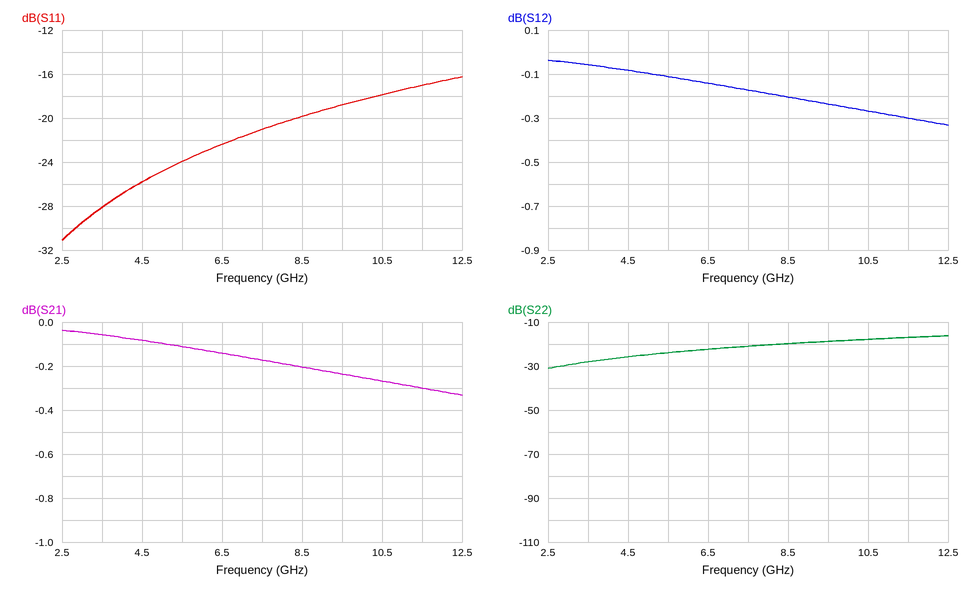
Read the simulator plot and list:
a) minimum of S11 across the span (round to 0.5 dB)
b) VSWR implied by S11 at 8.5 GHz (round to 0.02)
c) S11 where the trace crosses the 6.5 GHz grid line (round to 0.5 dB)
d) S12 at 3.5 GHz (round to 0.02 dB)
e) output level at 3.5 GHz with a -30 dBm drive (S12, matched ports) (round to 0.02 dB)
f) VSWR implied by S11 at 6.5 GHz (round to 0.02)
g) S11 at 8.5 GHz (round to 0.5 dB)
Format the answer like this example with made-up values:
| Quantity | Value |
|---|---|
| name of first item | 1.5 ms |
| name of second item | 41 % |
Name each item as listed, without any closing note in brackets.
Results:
| Quantity | Value |
|---|---|
| minimum of S11 across the span | -31.0 dB |
| VSWR implied by S11 at 8.5 GHz | 1.22 |
| S11 where the trace crosses the 6.5 GHz grid line | -22.5 dB |
| S12 at 3.5 GHz | -0.06 dB |
| output level at 3.5 GHz with a -30 dBm drive (S12, matched ports) | -30.06 dBm |
| VSWR implied by S11 at 6.5 GHz | 1.16 |
| S11 at 8.5 GHz | -20.0 dB |
